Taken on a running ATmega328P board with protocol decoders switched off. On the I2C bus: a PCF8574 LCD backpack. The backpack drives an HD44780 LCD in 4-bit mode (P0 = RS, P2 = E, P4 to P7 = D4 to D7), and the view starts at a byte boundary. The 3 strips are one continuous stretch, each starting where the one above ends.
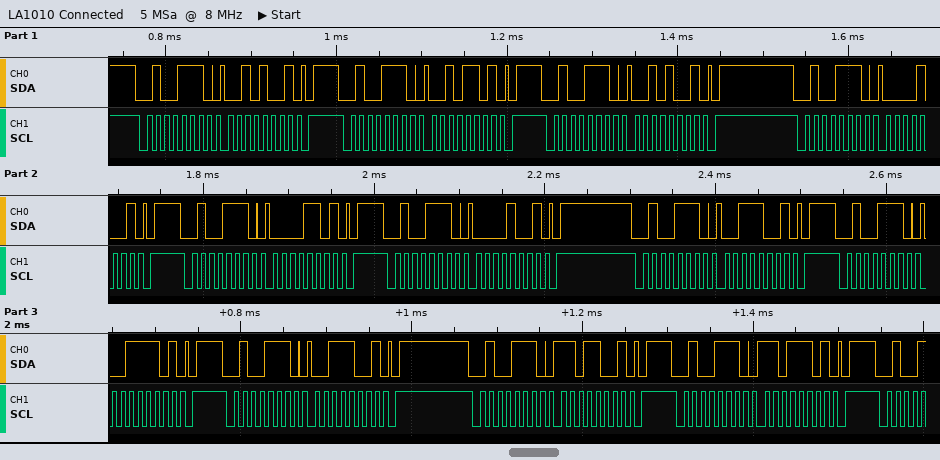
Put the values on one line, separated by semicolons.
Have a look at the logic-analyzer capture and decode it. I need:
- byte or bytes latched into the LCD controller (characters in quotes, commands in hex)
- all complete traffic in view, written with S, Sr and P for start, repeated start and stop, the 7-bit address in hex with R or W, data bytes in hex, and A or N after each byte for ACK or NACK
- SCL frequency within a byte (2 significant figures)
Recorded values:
' '; S 27W A 29 A P S 27W A 2D A P S 27W A 29 A P S 27W A 09 A P S 27W A 0D A P S 27W A 09 A P S 27W A 39 A P S 27W A 3D A P S 27W A 39 A P S 27W A D9 A P S 27W A DD A P; 100 kHz
